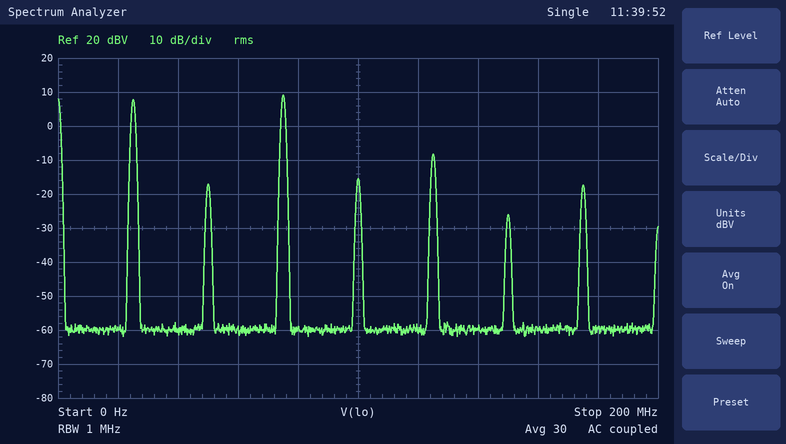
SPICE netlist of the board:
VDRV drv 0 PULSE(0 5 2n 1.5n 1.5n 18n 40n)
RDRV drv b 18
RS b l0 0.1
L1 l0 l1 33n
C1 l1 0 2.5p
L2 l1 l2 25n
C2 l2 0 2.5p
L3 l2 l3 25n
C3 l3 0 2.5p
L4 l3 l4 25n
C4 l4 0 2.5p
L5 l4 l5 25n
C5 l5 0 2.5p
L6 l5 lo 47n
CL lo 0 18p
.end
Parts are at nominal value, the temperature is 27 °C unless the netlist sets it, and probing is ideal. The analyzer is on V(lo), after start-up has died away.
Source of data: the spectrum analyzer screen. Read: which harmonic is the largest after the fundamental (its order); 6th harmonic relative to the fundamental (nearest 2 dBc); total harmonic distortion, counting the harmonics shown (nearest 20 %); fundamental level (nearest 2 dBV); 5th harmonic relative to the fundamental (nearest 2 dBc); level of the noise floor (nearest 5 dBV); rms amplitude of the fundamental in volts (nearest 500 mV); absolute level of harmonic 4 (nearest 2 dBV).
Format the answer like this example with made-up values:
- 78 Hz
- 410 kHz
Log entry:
- 3
- -34 dBc
- 120 %
- 8 dBV
- -16 dBc
- -60 dBV
- 2.5 V
- -16 dBV
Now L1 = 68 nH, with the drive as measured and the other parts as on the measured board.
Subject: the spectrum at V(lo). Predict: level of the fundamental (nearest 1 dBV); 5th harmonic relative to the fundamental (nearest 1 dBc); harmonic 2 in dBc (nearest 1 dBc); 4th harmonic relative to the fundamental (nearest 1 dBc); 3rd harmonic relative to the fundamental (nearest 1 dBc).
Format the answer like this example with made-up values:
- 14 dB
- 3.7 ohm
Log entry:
- 8 dBV
- -19 dBc
- -24 dBc
- -27 dBc
- 2 dBc
